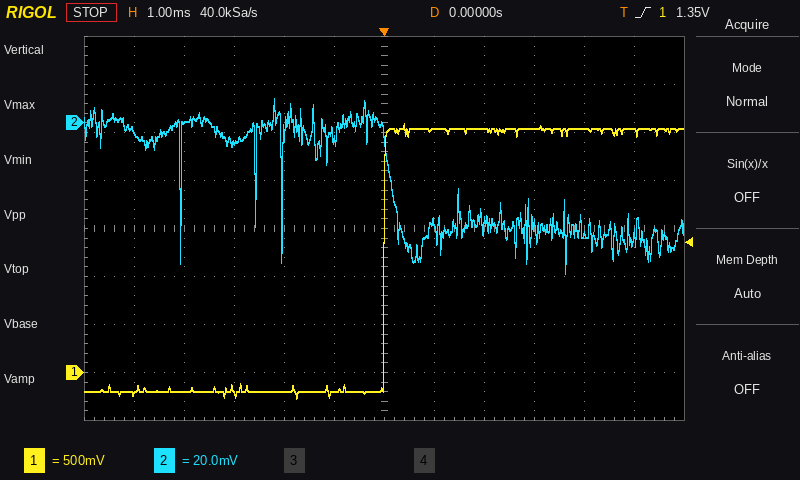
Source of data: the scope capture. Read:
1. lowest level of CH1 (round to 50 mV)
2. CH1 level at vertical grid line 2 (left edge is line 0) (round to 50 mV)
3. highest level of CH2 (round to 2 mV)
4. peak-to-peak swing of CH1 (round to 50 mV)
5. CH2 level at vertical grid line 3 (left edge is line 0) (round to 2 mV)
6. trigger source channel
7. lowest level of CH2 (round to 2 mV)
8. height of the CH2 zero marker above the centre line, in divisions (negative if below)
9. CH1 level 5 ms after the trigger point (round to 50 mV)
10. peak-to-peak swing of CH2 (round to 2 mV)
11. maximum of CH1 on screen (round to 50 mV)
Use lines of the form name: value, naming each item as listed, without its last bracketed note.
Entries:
lowest level of CH1: -250 mV
CH1 level at vertical grid line 2 (left edge is line 0): -200 mV
highest level of CH2: 10 mV
peak-to-peak swing of CH1: 2.85 V
CH2 level at vertical grid line 3 (left edge is line 0): -8 mV
trigger source channel: CH1
lowest level of CH2: -62 mV
height of the CH2 zero marker above the centre line, in divisions: +2.2 div
CH1 level 5 ms after the trigger point: 2.50 V
peak-to-peak swing of CH2: 72 mV
maximum of CH1 on screen: 2.60 V
